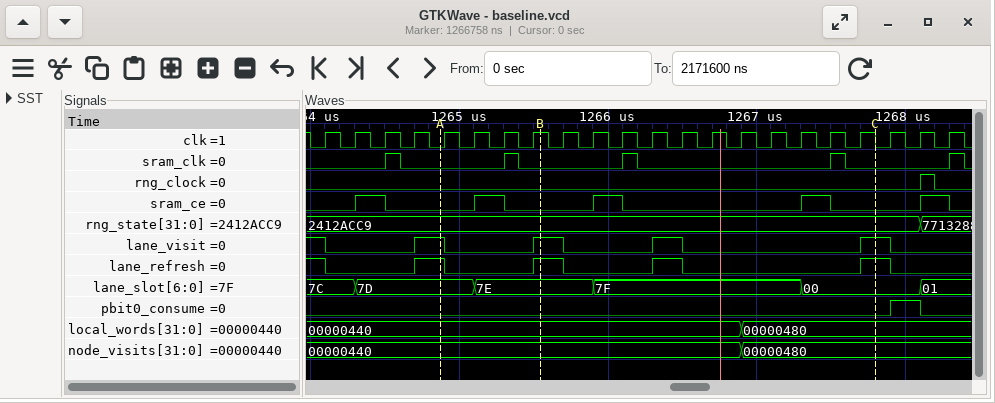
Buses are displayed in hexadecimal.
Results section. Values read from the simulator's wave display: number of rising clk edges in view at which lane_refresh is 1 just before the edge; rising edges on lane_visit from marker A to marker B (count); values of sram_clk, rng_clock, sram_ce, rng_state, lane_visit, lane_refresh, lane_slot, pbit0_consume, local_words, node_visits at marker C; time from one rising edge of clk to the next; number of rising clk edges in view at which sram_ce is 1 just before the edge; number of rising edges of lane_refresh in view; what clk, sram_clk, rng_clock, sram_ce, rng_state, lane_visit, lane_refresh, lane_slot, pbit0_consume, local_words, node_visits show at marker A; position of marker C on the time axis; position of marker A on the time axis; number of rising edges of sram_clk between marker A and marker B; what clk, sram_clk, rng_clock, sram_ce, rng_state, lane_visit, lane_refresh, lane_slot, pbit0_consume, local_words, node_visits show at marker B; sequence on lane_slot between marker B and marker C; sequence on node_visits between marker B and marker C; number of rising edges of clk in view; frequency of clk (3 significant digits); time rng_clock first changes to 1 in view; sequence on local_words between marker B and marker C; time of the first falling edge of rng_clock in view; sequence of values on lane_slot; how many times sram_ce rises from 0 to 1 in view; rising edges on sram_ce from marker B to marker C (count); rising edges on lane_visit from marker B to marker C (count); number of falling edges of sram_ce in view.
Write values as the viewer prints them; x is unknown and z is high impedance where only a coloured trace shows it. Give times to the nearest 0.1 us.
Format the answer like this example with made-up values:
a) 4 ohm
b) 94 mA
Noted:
a) 5
b) 1
c) sram_clk=0, rng_clock=0, sram_ce=0, rng_state=2412ACC9, lane_visit=1, lane_refresh=1, lane_slot=00, pbit0_consume=0, local_words=00000480, node_visits=00000480
d) 0.2 us
e) 5
f) 4
g) clk=0, sram_clk=0, rng_clock=0, sram_ce=0, rng_state=2412ACC9, lane_visit=1, lane_refresh=1, lane_slot=7D, pbit0_consume=0, local_words=00000440, node_visits=00000440
h) 1267.8 us
i) 1264.9 us
j) 1
k) clk=1, sram_clk=0, rng_clock=0, sram_ce=0, rng_state=2412ACC9, lane_visit=1, lane_refresh=1, lane_slot=7E, pbit0_consume=0, local_words=00000440, node_visits=00000440
l) 7E, 7F, 00
m) 00000440, 00000480
n) 22
o) 5.00 MHz
p) 1268.1 us
q) 00000440, 00000480
r) 1268.2 us
s) 7C, 7D, 7E, 7F, 00, 01
t) 5
u) 2
v) 2
w) 5
